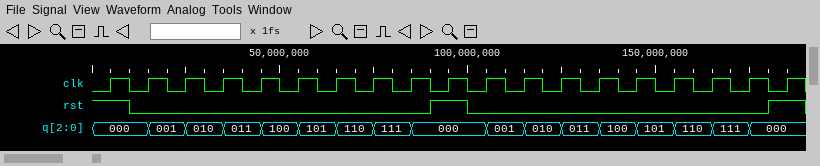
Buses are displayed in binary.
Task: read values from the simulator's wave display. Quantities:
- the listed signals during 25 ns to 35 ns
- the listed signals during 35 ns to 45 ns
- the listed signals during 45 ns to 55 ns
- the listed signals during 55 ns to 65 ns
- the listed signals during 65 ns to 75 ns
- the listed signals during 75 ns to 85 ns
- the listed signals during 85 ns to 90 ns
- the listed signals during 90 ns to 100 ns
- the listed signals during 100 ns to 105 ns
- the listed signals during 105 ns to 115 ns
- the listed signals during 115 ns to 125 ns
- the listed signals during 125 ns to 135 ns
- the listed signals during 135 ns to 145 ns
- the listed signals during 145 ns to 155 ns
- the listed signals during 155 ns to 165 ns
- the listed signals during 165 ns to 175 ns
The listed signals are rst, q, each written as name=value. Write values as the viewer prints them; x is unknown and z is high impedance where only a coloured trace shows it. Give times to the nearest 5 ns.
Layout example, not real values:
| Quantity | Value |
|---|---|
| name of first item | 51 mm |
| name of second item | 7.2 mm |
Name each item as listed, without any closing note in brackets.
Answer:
| Quantity | Value |
|---|---|
| the listed signals during 25 ns to 35 ns | rst=0, q=010 |
| the listed signals during 35 ns to 45 ns | rst=0, q=011 |
| the listed signals during 45 ns to 55 ns | rst=0, q=100 |
| the listed signals during 55 ns to 65 ns | rst=0, q=101 |
| the listed signals during 65 ns to 75 ns | rst=0, q=110 |
| the listed signals during 75 ns to 85 ns | rst=0, q=111 |
| the listed signals during 85 ns to 90 ns | rst=0, q=000 |
| the listed signals during 90 ns to 100 ns | rst=1, q=000 |
| the listed signals during 100 ns to 105 ns | rst=0, q=000 |
| the listed signals during 105 ns to 115 ns | rst=0, q=001 |
| the listed signals during 115 ns to 125 ns | rst=0, q=010 |
| the listed signals during 125 ns to 135 ns | rst=0, q=011 |
| the listed signals during 135 ns to 145 ns | rst=0, q=100 |
| the listed signals during 145 ns to 155 ns | rst=0, q=101 |
| the listed signals during 155 ns to 165 ns | rst=0, q=110 |
| the listed signals during 165 ns to 175 ns | rst=0, q=111 |
